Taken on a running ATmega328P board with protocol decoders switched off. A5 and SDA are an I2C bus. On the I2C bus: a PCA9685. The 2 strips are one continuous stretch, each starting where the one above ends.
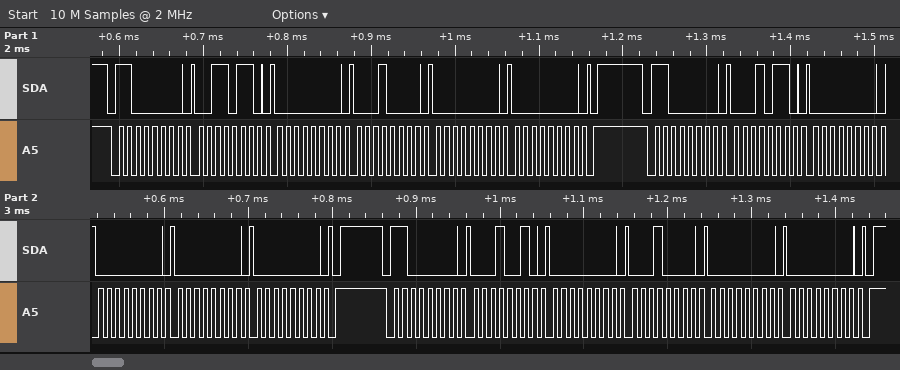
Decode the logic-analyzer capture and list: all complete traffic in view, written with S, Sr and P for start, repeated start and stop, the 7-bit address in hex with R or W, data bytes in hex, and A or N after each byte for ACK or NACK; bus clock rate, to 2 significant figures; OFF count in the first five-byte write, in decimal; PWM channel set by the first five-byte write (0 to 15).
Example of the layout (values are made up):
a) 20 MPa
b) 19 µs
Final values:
a) S 60W A 36 A 00 A 10 A 00 A 00 A P S 60W A 16 A 00 A 00 A 00 A 00 A P S 60W A 12 A 00 A 10 A 00 A 00 A P
b) 100 kHz
c) 0
d) 12
